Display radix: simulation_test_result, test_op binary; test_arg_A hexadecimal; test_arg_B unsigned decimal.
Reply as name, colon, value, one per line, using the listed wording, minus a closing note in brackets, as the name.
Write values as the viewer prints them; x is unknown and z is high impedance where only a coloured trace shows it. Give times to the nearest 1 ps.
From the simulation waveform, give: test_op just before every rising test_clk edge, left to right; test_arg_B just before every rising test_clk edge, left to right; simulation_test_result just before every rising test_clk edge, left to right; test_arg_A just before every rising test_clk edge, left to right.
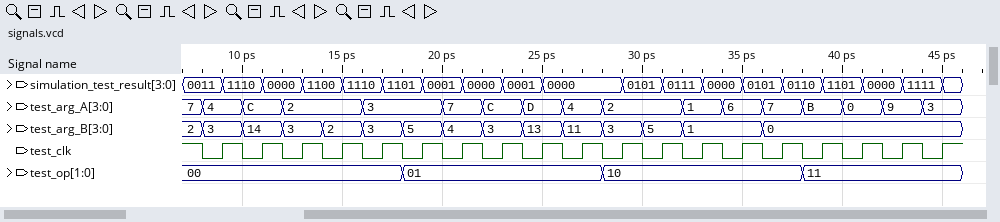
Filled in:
test_op just before every rising test_clk edge, left to right: 00, 00, 00, 00, 00, 01, 01, 01, 01, 01, 10, 10, 10, 10, 10, 11, 11, 11, 11
test_arg_B just before every rising test_clk edge, left to right: 3, 14, 3, 2, 3, 5, 4, 3, 13, 11, 3, 5, 1, 1, 0, 0, 0, 0, 0
simulation_test_result just before every rising test_clk edge, left to right: 0011, 1110, 0000, 1100, 1110, 1101, 0001, 0000, 0001, 0000, 0000, 0101, 0111, 0000, 0101, 0110, 1101, 0000, 1111
test_arg_A just before every rising test_clk edge, left to right: 4, C, 2, 2, 3, 3, 7, C, D, 4, 2, 2, 1, 6, 7, B, 0, 9, 3
